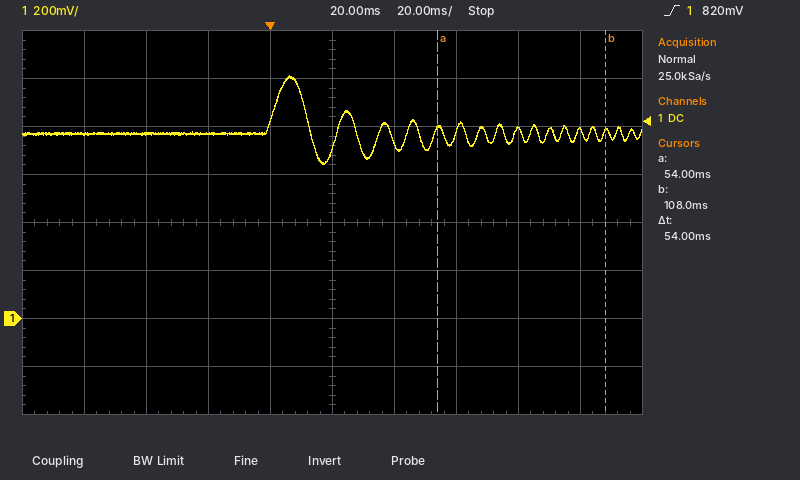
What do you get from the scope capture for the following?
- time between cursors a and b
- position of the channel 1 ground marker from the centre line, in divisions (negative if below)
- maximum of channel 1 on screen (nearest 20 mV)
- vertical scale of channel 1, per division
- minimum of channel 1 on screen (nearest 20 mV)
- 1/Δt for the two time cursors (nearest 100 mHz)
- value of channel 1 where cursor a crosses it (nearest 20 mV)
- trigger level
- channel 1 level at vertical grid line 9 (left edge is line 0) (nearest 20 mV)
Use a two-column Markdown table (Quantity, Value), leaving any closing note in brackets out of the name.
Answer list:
| Quantity | Value |
|---|---|
| time between cursors a and b | 54 ms |
| position of the channel 1 ground marker from the centre line, in divisions | -2.0 div |
| maximum of channel 1 on screen | 1.02 V |
| vertical scale of channel 1, per division | 200 mV |
| minimum of channel 1 on screen | 640 mV |
| 1/Δt for the two time cursors | 18.5 Hz |
| value of channel 1 where cursor a crosses it | 780 mV |
| trigger level | 820 mV |
| channel 1 level at vertical grid line 9 (left edge is line 0) | 780 mV |
